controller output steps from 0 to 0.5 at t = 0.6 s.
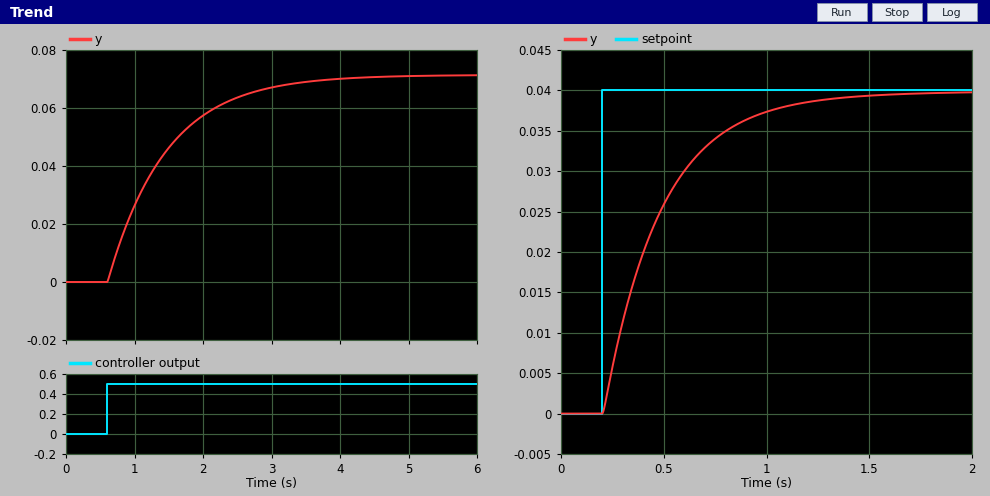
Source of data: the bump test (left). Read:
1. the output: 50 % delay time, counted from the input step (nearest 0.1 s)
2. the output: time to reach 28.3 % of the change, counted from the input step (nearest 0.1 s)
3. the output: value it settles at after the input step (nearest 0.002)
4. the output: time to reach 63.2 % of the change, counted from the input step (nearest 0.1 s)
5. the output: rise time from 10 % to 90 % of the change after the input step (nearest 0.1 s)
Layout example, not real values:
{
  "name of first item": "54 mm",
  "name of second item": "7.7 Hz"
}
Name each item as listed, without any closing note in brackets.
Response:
{
  "the output: 50 % delay time, counted from the input step": "0.6 s",
  "the output: time to reach 28.3 % of the change, counted from the input step": "0.3 s",
  "the output: value it settles at after the input step": "0.072",
  "the output: time to reach 63.2 % of the change, counted from the input step": "0.9 s",
  "the output: rise time from 10 % to 90 % of the change after the input step": "1.9 s"
}
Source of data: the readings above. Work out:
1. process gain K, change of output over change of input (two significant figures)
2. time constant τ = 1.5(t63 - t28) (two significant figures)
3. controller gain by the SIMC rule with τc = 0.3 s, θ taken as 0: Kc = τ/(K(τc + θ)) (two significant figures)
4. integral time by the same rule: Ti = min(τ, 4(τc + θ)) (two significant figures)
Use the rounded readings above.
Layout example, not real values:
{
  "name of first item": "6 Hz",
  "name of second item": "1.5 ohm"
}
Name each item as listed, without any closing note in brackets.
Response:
{
  "process gain K, change of output over change of input": "0.14",
  "time constant τ = 1.5(t63 - t28)": "0.90 s",
  "controller gain by the SIMC rule with τc = 0.3 s, θ taken as 0: Kc = τ/(K(τc + θ))": "21",
  "integral time by the same rule: Ti = min(τ, 4(τc + θ))": "0.90 s"
}
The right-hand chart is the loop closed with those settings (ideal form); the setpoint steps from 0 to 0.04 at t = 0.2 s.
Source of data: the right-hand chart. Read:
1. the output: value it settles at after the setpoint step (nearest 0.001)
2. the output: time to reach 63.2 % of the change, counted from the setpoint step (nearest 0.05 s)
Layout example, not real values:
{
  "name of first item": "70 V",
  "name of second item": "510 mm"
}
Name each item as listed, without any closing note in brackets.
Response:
{
  "the output: value it settles at after the setpoint step": "0.040",
  "the output: time to reach 63.2 % of the change, counted from the setpoint step": "0.30 s"
}
